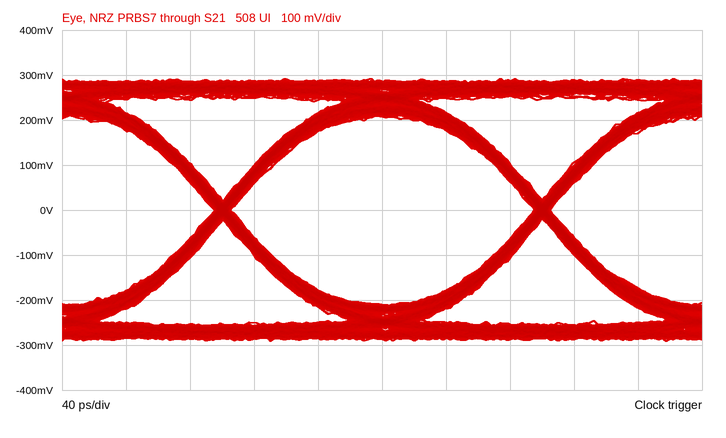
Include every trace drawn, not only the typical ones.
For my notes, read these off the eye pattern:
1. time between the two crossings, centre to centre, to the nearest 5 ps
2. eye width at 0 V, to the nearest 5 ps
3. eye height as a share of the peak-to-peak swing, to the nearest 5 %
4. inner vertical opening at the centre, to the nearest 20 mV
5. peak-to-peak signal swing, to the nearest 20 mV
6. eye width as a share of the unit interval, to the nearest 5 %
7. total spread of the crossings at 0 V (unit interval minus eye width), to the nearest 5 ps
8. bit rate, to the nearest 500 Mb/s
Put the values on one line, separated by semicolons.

200 ps; 190 ps; 70 %; 420 mV; 580 mV; 95 %; 10 ps; 5.0 Gb/s
